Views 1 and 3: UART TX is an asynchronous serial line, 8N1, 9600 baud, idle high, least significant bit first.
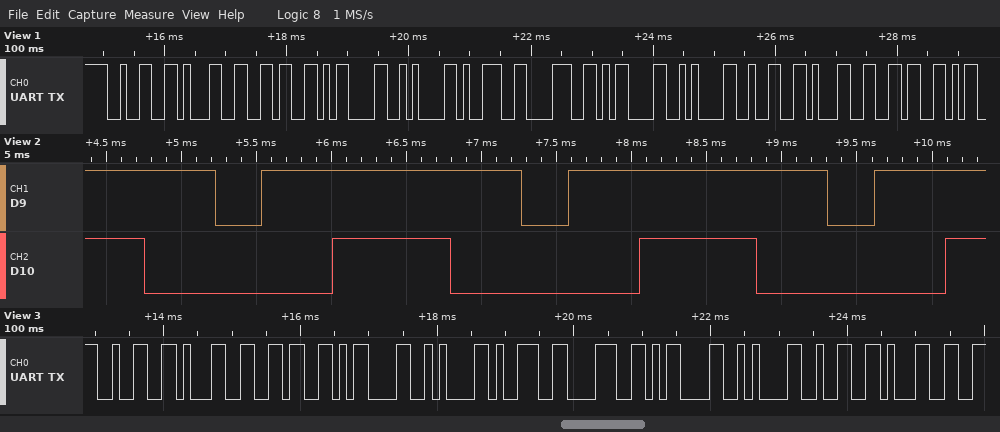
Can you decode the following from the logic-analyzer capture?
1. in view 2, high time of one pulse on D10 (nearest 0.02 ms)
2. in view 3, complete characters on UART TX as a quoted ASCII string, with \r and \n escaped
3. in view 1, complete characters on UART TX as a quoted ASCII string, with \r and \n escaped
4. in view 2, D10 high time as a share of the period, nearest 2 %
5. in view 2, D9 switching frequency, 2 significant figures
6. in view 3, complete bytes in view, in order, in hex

0.78 ms
"216\r\n98\r\n21"
"216\r\n98\r\n216"
38 %
490 Hz
32 31 36 0D 0A 39 38 0D 0A 32 31
